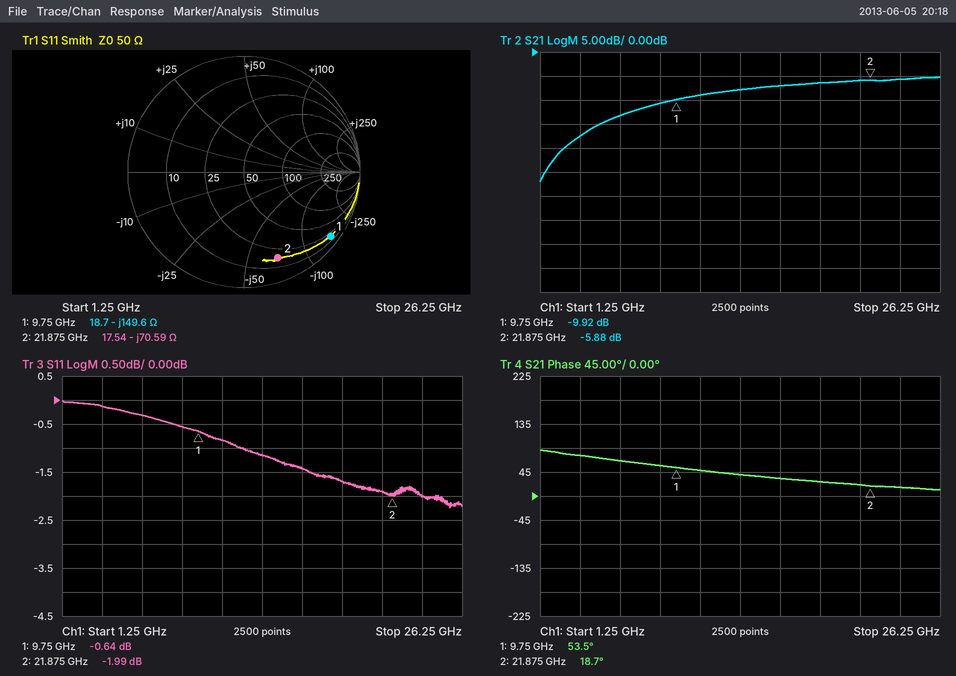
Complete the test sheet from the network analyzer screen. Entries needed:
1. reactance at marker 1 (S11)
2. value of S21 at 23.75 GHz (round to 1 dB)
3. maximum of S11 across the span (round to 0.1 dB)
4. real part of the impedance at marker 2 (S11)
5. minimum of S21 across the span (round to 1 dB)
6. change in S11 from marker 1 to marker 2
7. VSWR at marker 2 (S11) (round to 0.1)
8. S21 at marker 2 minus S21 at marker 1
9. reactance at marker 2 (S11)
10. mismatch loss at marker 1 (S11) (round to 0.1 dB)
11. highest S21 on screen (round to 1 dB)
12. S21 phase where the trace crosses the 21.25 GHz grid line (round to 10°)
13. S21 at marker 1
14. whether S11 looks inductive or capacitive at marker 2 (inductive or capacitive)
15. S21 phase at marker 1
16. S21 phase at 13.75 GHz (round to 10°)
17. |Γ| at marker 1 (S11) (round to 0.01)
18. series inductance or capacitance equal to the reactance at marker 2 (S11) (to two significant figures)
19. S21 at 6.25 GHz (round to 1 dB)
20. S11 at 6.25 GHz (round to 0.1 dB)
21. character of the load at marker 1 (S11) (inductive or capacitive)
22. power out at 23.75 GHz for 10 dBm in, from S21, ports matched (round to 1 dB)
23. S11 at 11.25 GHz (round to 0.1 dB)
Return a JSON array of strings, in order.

["-149.6 Ω", "-6 dB", "0.0 dB", "17.54 Ω", "-27 dB", "-1.35 dB", "8.8", "4.04 dB", "-70.59 Ω", "8.6 dB", "-5 dB", "20°", "-9.92 dB", "capacitive", "53.5°", "40°", "0.93", "100 fF", "-13 dB", "-0.3 dB", "capacitive", "4 dBm", "-0.8 dB"]
